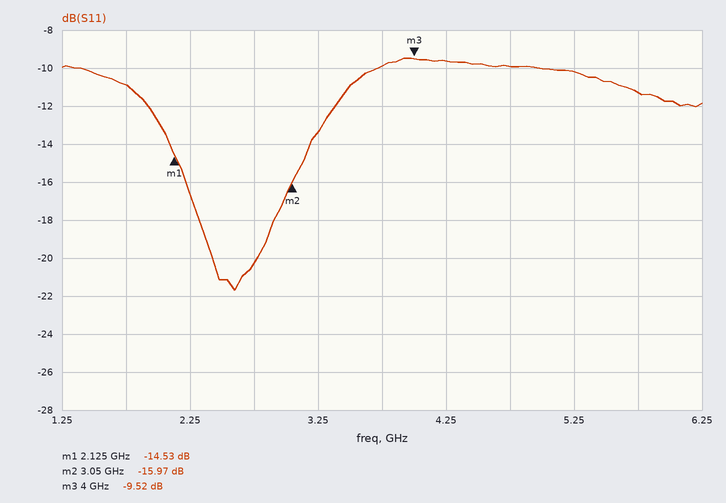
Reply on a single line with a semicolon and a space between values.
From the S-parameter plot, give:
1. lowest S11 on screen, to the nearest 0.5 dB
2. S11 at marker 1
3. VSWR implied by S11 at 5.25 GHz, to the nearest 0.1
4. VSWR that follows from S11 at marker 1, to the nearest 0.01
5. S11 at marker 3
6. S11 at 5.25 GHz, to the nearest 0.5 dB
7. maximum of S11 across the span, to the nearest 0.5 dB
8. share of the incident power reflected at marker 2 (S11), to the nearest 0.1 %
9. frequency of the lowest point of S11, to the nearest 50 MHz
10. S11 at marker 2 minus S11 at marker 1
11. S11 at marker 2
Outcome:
-21.5 dB; -14.53 dB; 1.9; 1.46; -9.52 dB; -10.0 dB; -9.5 dB; 2.5 %; 2.60 GHz; -1.44 dB; -15.97 dB
